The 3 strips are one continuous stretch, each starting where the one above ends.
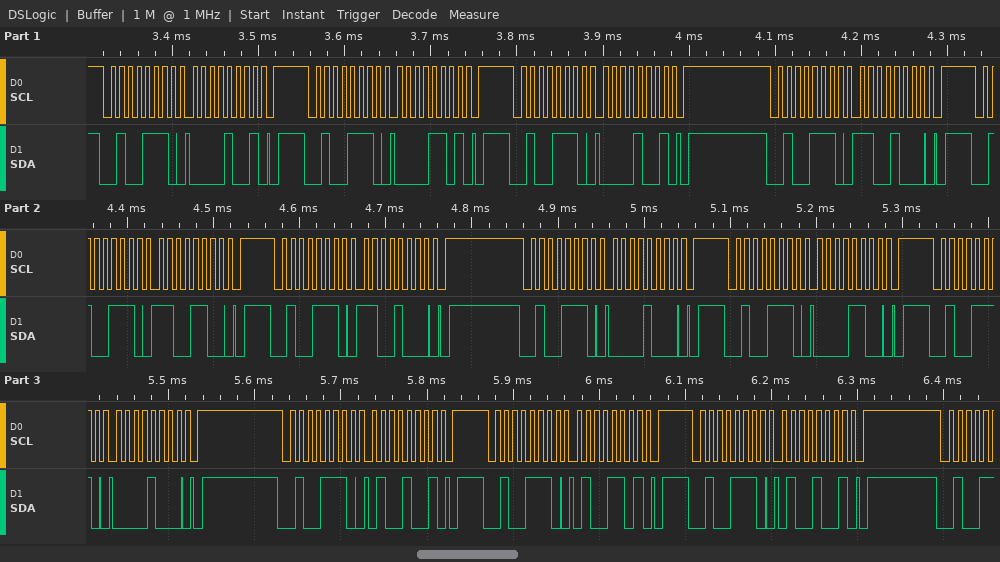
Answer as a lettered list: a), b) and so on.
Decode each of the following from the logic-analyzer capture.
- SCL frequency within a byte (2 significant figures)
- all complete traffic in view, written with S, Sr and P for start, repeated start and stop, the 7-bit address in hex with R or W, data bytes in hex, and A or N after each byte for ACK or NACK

a) 100 kHz
b) S 27W A 09 A P S 27W A 0D A P S 27W A 09 A P S 27W A C8 A P S 27W A CC A P S 27W A C8 A P S 27W A 08 A P S 27W A 0C A P S 27W A 08 A P S 27W A 49 A P S 27W A 4D A P S 27W A 49 A P
